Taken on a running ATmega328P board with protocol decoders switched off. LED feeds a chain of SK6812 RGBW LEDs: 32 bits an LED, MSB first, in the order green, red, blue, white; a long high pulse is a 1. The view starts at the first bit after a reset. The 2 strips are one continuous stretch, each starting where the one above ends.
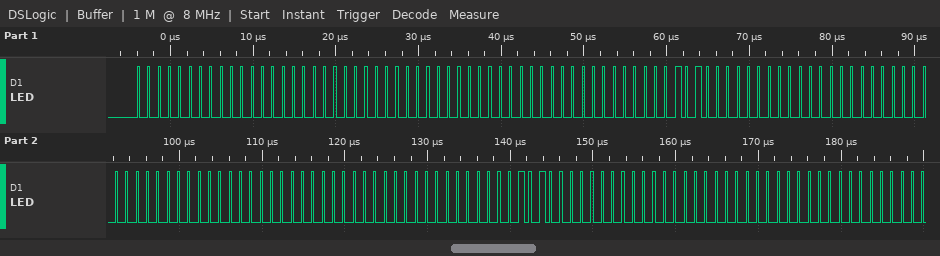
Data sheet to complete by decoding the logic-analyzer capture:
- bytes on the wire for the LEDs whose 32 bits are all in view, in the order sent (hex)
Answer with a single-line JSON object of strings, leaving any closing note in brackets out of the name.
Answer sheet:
{"bytes on the wire for the LEDs whose 32 bits are all in view, in the order sent": "00 00 00 00 00 00 0A 00 00 00 00 00 00 00 0A 00"}
